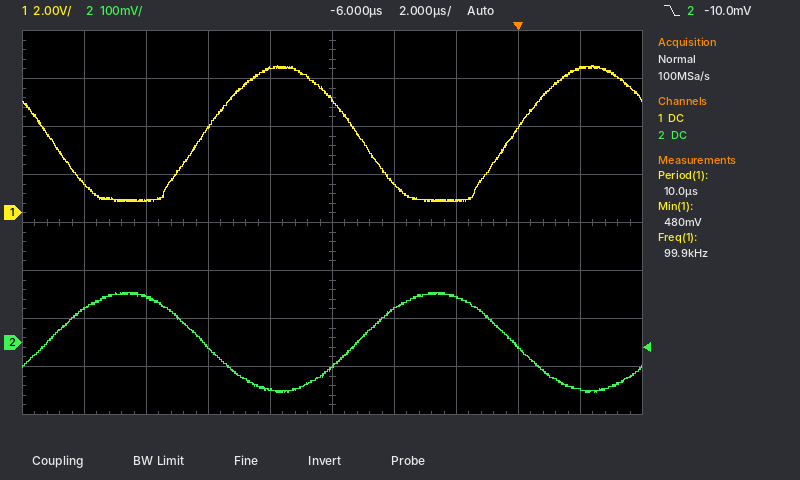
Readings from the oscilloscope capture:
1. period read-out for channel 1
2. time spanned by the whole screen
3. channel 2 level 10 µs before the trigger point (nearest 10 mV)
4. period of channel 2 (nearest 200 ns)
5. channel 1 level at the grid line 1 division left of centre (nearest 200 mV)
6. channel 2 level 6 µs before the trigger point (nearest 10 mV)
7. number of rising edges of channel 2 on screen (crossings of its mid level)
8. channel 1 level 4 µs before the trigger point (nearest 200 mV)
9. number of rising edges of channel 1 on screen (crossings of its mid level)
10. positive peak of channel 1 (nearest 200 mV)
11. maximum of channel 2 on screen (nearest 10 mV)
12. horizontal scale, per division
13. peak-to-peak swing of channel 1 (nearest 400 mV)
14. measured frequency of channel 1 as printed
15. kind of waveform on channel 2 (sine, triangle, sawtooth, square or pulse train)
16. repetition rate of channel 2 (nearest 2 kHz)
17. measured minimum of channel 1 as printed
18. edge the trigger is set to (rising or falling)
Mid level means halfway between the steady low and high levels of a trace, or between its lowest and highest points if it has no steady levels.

10.0 µs
20 µs
-10 mV
10.0 µs
6.0 V
-50 mV
2
1.2 V
2
6.2 V
100 mV
2 µs
5.6 V
99.9 kHz
sine
100 kHz
480 mV
falling
